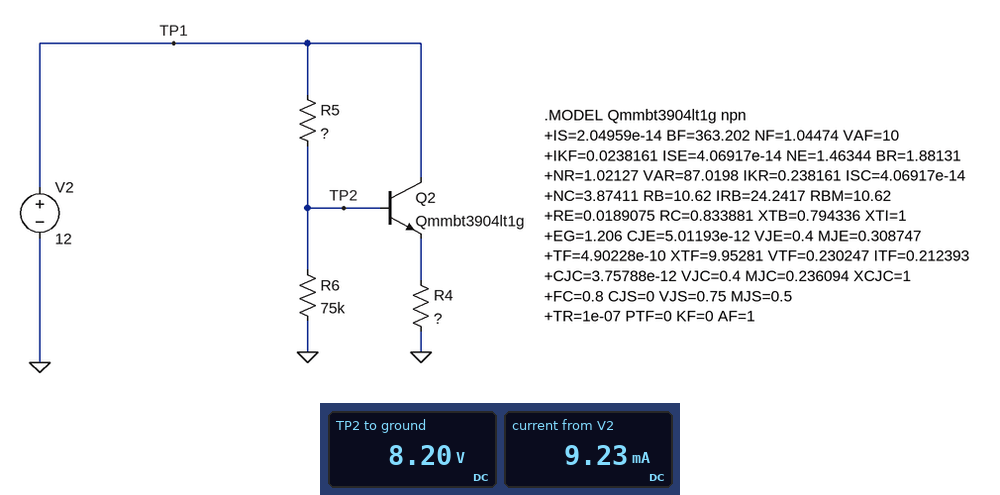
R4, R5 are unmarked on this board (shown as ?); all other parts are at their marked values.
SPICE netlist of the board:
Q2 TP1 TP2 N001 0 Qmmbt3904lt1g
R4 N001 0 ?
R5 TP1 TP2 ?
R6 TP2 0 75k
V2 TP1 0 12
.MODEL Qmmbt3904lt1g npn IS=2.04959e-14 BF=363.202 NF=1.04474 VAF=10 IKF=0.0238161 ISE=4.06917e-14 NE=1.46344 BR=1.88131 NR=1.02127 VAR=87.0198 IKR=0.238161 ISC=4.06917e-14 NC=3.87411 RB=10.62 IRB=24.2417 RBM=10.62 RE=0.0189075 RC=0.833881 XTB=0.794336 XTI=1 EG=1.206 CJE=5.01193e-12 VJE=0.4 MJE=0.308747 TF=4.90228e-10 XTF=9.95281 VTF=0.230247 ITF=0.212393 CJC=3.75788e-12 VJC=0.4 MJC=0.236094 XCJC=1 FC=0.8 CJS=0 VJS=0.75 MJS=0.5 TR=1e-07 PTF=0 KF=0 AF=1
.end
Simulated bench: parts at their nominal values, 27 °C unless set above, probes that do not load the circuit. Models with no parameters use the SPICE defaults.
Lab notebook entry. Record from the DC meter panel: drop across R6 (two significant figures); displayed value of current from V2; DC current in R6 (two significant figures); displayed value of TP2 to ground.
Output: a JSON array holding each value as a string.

["8.2 V", "9.23 mA", "110 µA", "8.20 V"]
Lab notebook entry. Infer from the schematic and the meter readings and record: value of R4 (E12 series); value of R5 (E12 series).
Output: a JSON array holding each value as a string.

["820 Ω", "27 kΩ"]
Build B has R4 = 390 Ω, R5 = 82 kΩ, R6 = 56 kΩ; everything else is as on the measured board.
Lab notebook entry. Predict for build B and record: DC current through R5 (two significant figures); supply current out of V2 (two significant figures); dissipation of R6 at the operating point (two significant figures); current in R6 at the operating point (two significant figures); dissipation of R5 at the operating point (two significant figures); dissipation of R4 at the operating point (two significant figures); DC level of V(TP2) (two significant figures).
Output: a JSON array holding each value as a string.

["96 µA", "8.8 mA", "300 µW", "74 µA", "760 µW", "30 mW", "4.1 V"]
